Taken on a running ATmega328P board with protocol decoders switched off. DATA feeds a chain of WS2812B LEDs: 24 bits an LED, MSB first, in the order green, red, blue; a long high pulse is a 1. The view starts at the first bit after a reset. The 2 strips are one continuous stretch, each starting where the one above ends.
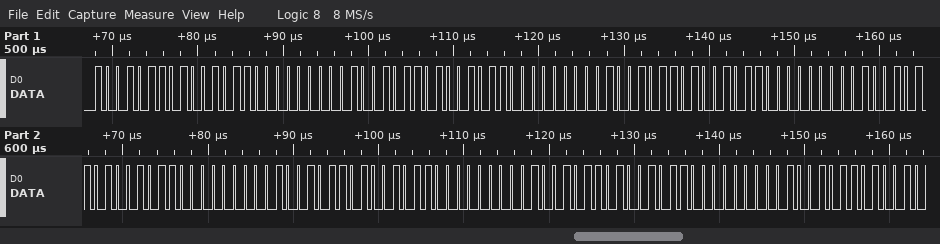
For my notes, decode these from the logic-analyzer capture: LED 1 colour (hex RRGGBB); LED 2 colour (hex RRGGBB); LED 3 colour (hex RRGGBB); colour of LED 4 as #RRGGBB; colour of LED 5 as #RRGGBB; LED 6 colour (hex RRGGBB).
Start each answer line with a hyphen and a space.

- #969600
- #969600
- #969600
- #969600
- #969600
- #969600
